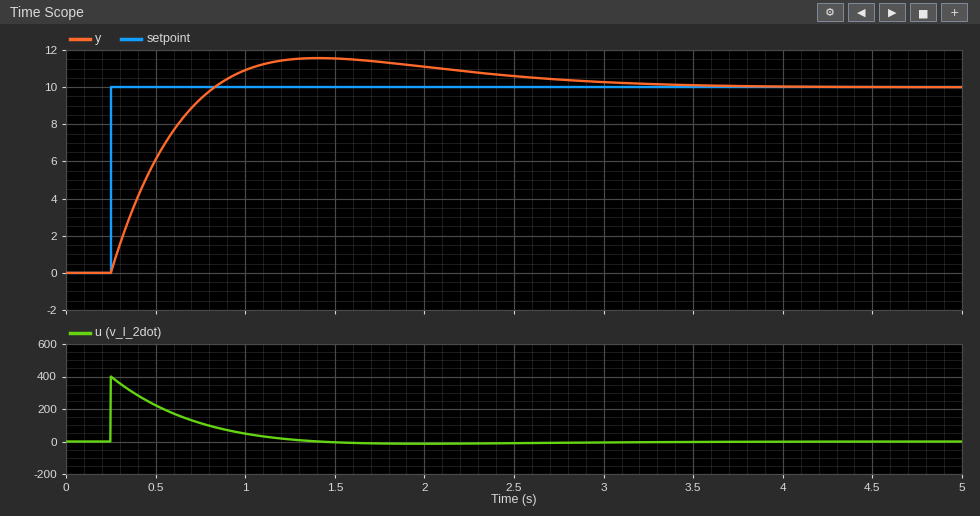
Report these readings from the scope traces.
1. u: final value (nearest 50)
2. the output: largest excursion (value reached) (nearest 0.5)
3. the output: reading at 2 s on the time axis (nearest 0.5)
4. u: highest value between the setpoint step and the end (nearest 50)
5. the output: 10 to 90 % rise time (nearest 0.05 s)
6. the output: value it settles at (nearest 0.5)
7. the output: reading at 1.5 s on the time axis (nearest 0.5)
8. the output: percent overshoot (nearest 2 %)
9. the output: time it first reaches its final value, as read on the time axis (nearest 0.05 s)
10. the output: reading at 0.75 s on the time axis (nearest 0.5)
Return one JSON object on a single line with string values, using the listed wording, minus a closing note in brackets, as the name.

{"u: final value": "0", "the output: largest excursion (value reached)": "11.5", "the output: reading at 2 s on the time axis": "11.0", "u: highest value between the setpoint step and the end": "400", "the output: 10 to 90 % rise time": "0.45 s", "the output: value it settles at": "10.0", "the output: reading at 1.5 s on the time axis": "11.5", "the output: percent overshoot": "16 %", "the output: time it first reaches its final value, as read on the time axis": "0.85 s", "the output: reading at 0.75 s on the time axis": "9.5"}
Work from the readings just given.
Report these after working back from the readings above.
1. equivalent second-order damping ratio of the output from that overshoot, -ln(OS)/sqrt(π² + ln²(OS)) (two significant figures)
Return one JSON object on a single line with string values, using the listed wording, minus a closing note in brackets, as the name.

{"equivalent second-order damping ratio of the output from that overshoot, -ln(OS)/sqrt(π² + ln²(OS))": "0.50"}
